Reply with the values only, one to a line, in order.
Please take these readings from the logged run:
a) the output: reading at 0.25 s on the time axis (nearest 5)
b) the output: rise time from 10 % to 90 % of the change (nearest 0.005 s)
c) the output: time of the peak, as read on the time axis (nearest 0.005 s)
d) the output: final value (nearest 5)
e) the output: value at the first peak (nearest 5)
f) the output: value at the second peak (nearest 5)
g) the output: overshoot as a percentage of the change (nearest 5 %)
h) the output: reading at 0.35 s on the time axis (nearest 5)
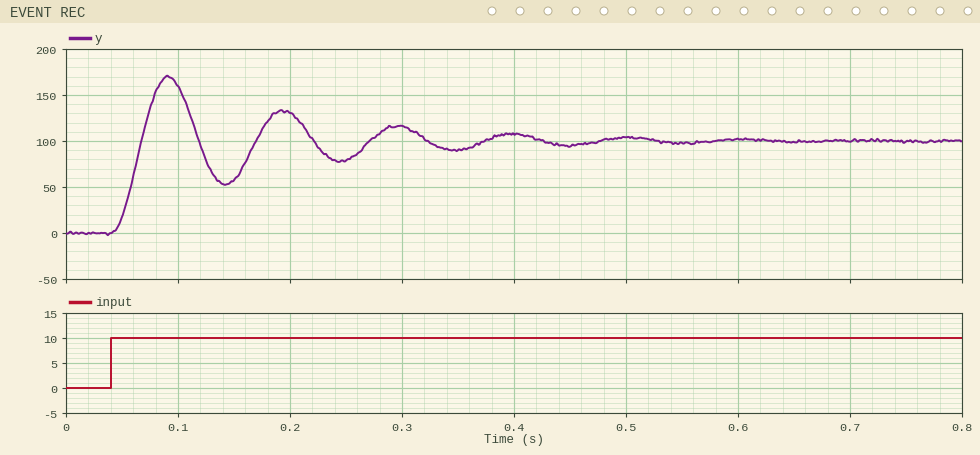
80
0.020 s
0.090 s
100
170
135
70 %
90
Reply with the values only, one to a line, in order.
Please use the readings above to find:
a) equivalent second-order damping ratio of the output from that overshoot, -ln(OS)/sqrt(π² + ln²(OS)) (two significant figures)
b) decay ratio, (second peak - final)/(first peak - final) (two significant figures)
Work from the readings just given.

0.11
0.50
